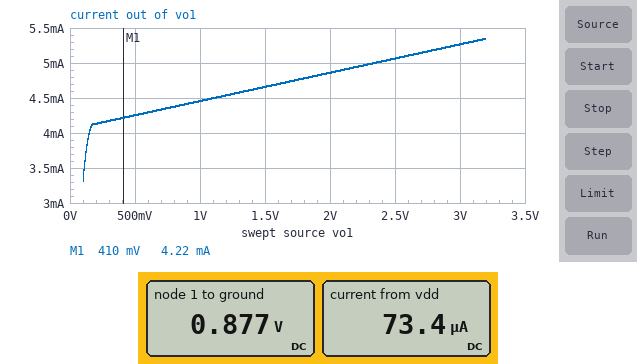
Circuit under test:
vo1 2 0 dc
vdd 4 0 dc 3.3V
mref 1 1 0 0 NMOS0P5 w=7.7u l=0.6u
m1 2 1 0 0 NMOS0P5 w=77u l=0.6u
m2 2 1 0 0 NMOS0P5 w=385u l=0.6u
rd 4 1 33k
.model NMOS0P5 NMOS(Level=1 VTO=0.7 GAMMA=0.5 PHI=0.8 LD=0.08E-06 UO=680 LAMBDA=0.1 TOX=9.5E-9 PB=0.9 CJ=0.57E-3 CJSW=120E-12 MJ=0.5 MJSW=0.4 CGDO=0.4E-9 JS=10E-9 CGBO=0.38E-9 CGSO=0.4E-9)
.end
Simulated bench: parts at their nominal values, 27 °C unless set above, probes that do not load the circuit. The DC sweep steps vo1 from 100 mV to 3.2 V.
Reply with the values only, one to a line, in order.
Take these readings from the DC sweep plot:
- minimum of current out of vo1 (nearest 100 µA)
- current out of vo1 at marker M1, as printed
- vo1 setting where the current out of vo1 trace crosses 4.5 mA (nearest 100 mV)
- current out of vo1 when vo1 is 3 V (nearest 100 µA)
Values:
3.3 mA
4.22 mA
1.1 V
5.3 mA
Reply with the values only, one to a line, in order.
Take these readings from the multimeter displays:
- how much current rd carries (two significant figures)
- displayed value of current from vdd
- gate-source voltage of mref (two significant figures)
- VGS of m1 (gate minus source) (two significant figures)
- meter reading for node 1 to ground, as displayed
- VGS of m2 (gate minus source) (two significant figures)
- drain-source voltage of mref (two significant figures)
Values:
73 µA
73.4 µA
880 mV
880 mV
0.877 V
880 mV
880 mV
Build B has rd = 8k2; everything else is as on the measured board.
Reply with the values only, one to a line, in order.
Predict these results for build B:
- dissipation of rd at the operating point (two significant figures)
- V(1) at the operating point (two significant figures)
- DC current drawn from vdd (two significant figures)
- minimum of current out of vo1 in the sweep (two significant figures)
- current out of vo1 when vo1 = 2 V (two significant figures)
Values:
620 µW
1.0 V
280 µA
7.6 mA
18 mA
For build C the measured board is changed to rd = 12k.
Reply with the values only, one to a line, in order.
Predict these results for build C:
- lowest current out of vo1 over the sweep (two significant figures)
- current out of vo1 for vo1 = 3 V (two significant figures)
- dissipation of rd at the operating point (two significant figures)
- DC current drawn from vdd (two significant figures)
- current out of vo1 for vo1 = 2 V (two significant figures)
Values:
6.2 mA
14 mA
450 µW
190 µA
13 mA
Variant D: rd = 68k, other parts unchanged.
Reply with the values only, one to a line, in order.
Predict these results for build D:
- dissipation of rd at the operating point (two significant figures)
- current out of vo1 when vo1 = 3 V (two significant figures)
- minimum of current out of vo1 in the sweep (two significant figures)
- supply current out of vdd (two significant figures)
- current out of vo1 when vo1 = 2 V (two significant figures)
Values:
90 µW
2.6 mA
2.0 mA
36 µA
2.4 mA
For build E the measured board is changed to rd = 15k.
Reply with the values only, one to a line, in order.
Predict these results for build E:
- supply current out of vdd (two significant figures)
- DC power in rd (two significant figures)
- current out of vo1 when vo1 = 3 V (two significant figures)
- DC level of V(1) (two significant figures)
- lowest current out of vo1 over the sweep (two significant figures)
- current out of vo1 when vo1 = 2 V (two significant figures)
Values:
160 µA
370 µW
11 mA
960 mV
5.4 mA
10 mA
